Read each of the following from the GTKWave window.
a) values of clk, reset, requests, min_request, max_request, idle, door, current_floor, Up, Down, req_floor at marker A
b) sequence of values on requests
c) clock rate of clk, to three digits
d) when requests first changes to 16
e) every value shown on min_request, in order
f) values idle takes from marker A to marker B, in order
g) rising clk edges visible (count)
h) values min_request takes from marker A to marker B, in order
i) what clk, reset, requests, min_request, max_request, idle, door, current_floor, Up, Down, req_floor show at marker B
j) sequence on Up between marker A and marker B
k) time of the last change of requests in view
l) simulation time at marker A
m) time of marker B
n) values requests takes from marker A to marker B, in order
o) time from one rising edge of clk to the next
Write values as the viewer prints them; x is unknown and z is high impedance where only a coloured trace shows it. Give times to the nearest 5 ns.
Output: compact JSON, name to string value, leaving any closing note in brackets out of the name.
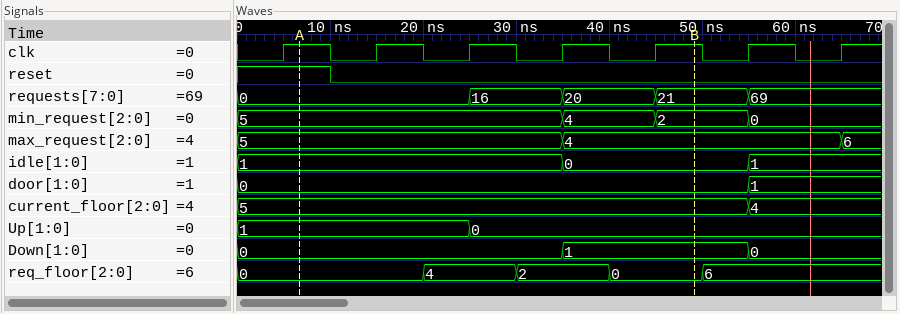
{"values of clk, reset, requests, min_request, max_request, idle, door, current_floor, Up, Down, req_floor at marker A": "clk=1, reset=1, requests=0, min_request=5, max_request=5, idle=1, door=0, current_floor=5, Up=1, Down=0, req_floor=0", "sequence of values on requests": "0, 16, 20, 21, 69", "clock rate of clk, to three digits": "100 MHz", "when requests first changes to 16": "25 ns", "every value shown on min_request, in order": "5, 4, 2, 0", "values idle takes from marker A to marker B, in order": "1, 0", "rising clk edges visible": "7", "values min_request takes from marker A to marker B, in order": "5, 4, 2", "what clk, reset, requests, min_request, max_request, idle, door, current_floor, Up, Down, req_floor show at marker B": "clk=1, reset=0, requests=21, min_request=2, max_request=4, idle=0, door=0, current_floor=5, Up=0, Down=1, req_floor=0", "sequence on Up between marker A and marker B": "1, 0", "time of the last change of requests in view": "55 ns", "simulation time at marker A": "5 ns", "time of marker B": "50 ns", "values requests takes from marker A to marker B, in order": "0, 16, 20, 21", "time from one rising edge of clk to the next": "10 ns"}
